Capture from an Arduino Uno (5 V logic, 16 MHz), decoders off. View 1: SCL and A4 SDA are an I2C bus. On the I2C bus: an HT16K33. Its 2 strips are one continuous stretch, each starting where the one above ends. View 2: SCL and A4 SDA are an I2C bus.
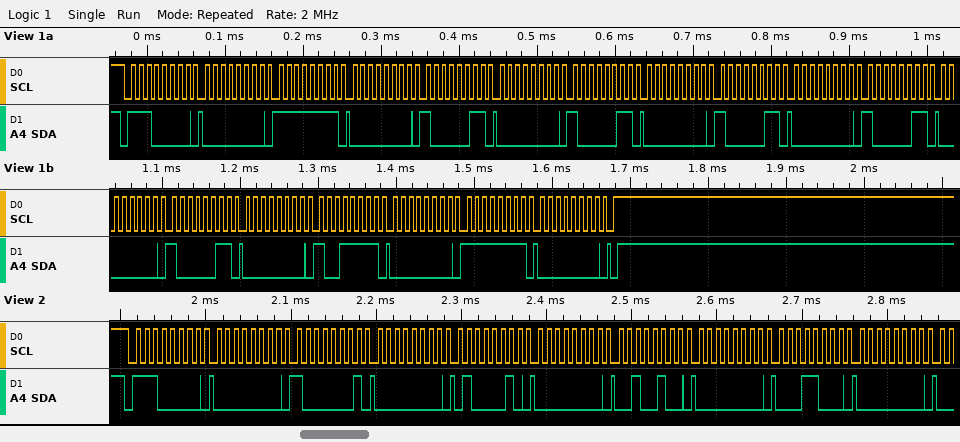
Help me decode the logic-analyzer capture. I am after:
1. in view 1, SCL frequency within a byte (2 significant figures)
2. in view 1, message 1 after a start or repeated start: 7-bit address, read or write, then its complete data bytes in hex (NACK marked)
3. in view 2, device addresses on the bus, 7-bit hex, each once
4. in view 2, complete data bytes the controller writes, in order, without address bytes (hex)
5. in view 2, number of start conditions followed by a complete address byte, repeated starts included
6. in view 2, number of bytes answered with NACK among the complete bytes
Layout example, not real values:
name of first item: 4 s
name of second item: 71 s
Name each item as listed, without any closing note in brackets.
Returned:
in view 1, SCL frequency within a byte: 100 kHz
in view 1, message 1 after a start or repeated start: 7-bit address, read or write, then its complete data bytes in hex: 0x70 write: 00 FF 00 83 00 83 00 83 00 83 00 83 00 9F 00 FF 00
in view 2, device addresses on the bus, 7-bit hex, each once: 0x70
in view 2, complete data bytes the controller writes, in order, without address bytes: 00 81 00 42 00 24 00 18 00
in view 2, number of start conditions followed by a complete address byte, repeated starts included: 1
in view 2, number of bytes answered with NACK among the complete bytes: 0
